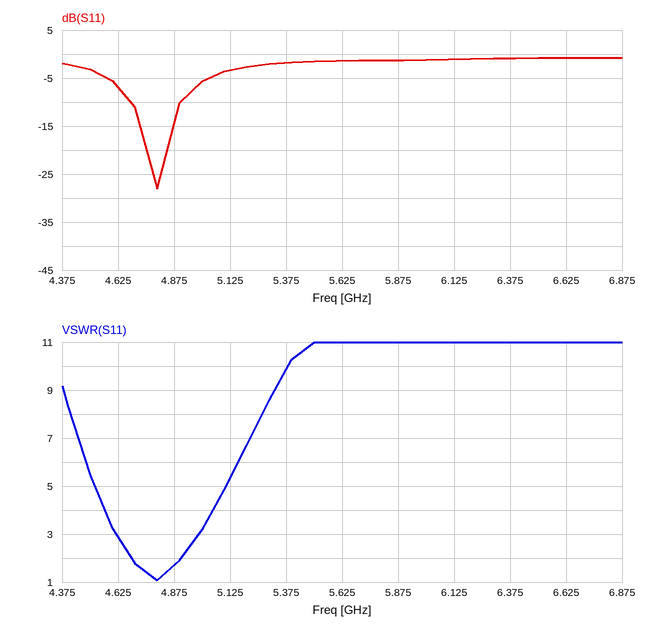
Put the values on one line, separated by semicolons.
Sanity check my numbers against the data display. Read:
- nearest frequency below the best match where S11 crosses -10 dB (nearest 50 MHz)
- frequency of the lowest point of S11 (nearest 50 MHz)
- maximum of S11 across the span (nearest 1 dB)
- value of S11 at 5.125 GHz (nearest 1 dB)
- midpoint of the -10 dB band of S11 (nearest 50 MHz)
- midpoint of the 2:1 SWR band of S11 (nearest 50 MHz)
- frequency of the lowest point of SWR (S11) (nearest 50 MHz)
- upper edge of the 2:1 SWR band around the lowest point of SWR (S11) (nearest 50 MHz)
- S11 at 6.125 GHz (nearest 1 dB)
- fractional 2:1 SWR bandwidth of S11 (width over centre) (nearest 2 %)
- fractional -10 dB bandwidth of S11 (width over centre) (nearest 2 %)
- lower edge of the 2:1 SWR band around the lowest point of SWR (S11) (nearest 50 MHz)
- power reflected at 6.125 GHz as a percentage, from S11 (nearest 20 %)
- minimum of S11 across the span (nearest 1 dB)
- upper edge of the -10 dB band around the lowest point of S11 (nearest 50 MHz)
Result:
4.70 GHz; 4.80 GHz; -1 dB; -3 dB; 4.80 GHz; 4.80 GHz; 4.80 GHz; 4.90 GHz; -1 dB; 4 %; 4 %; 4.70 GHz; 80 %; -28 dB; 4.90 GHz
